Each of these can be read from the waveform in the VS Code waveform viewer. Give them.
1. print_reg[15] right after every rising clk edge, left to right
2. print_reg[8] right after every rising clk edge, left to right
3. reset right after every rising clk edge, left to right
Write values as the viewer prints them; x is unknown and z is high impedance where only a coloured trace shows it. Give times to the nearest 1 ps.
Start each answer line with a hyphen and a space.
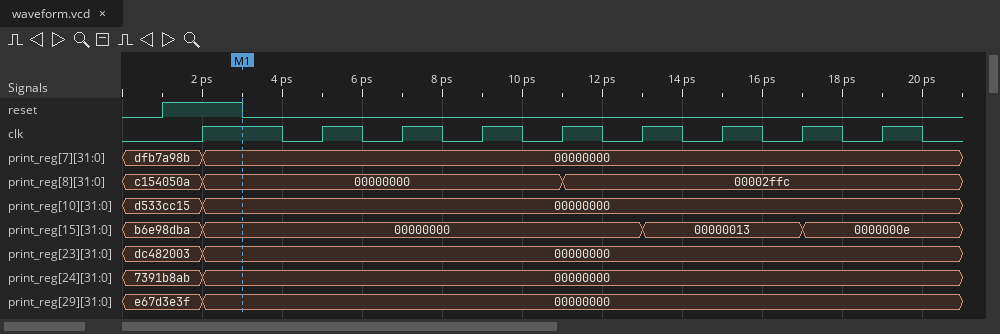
- 00000000, 00000000, 00000000, 00000000, 00000000, 00000013, 00000013, 0000000e, 0000000e
- 00000000, 00000000, 00000000, 00000000, 00002ffc, 00002ffc, 00002ffc, 00002ffc, 00002ffc
- 1 0 0 0 0 0 0 0 0
